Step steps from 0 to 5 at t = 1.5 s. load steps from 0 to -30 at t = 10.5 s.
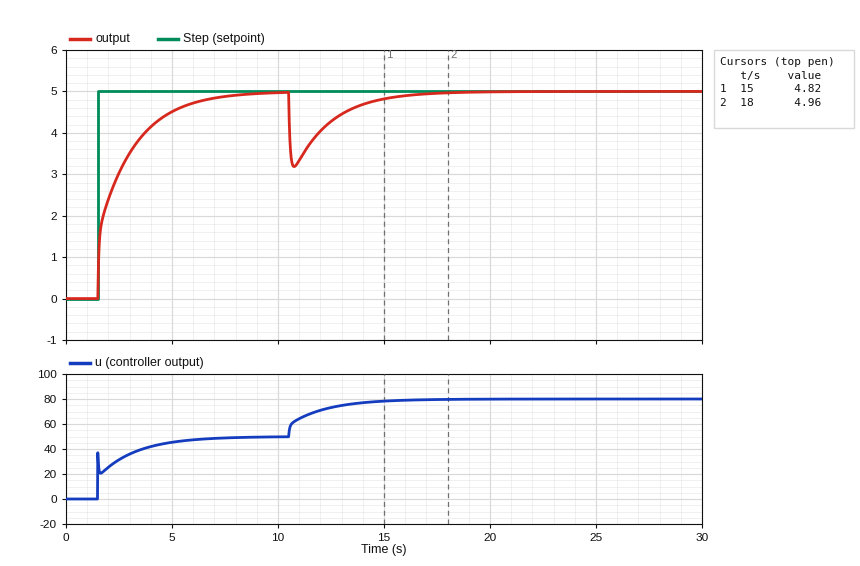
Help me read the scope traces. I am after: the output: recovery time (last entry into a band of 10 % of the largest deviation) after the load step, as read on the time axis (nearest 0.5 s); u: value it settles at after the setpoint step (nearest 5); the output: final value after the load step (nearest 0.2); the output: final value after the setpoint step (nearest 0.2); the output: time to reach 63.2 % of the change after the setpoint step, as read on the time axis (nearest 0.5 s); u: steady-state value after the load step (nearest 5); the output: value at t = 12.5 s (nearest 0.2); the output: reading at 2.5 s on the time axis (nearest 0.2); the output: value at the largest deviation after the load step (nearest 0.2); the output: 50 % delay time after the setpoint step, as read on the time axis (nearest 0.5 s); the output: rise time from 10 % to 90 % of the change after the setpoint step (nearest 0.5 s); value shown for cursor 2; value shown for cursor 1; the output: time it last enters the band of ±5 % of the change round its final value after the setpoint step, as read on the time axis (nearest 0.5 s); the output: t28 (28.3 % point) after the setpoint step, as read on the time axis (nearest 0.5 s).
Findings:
15.0 s
50
5.0
5.0
2.5 s
80
4.2
3.0
3.2
2.0 s
3.5 s
4.96
4.82
6.0 s
1.5 s
